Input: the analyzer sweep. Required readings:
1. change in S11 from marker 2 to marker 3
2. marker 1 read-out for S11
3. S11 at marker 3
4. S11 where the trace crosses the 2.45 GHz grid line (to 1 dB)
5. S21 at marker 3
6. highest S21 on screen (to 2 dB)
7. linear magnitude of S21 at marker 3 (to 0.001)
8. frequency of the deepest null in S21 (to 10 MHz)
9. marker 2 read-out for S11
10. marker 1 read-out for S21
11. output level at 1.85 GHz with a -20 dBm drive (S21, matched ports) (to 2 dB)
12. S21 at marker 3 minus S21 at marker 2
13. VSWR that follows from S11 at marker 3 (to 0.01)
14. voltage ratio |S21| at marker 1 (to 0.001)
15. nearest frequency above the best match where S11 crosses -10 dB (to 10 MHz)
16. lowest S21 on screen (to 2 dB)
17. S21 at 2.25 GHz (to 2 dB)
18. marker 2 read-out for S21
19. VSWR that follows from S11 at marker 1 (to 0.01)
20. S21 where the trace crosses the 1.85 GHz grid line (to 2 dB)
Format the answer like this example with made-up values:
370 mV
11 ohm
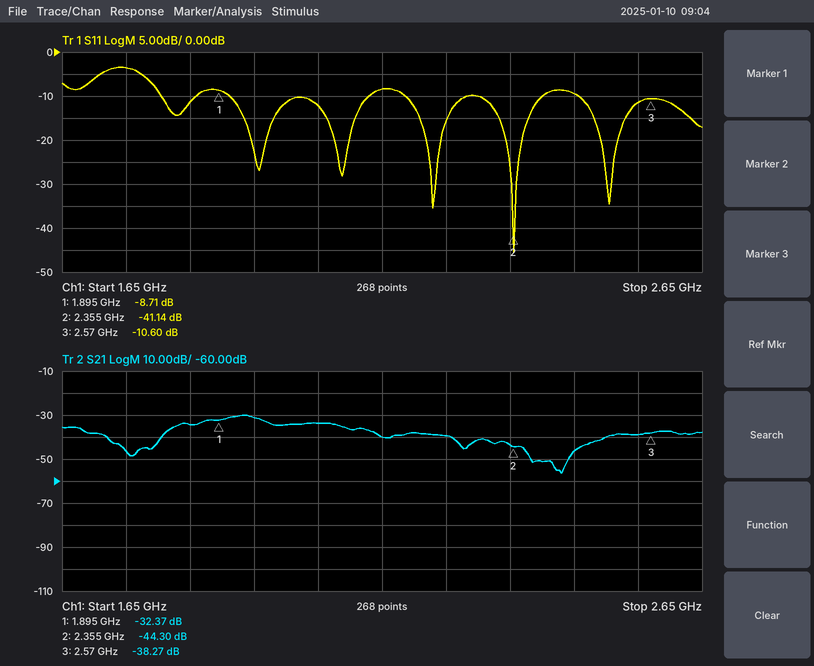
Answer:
30.54 dB
-8.71 dB
-10.60 dB
-9 dB
-38.27 dB
-30 dB
0.012
2.43 GHz
-41.14 dB
-32.37 dB
-54 dBm
6.03 dB
1.84
0.024
2.40 GHz
-56 dB
-40 dB
-44.30 dB
2.16
-34 dB
